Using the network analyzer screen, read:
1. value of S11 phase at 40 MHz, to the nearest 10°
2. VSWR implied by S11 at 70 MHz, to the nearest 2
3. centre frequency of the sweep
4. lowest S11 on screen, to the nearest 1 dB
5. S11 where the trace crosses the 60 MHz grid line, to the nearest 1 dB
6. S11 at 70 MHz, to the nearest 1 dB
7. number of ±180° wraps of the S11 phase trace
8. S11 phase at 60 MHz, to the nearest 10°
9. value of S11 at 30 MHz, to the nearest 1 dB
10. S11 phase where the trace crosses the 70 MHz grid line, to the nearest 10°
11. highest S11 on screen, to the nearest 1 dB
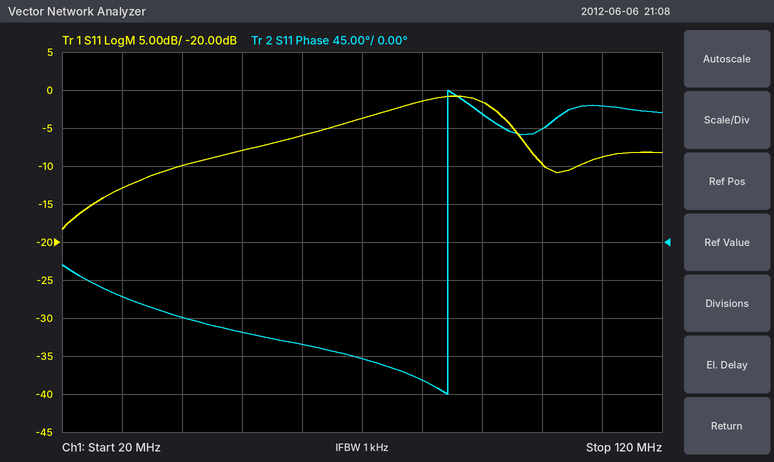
-90°
4
70 MHz
-18 dB
-6 dB
-4 dB
1
-120°
-13 dB
-140°
-1 dB
